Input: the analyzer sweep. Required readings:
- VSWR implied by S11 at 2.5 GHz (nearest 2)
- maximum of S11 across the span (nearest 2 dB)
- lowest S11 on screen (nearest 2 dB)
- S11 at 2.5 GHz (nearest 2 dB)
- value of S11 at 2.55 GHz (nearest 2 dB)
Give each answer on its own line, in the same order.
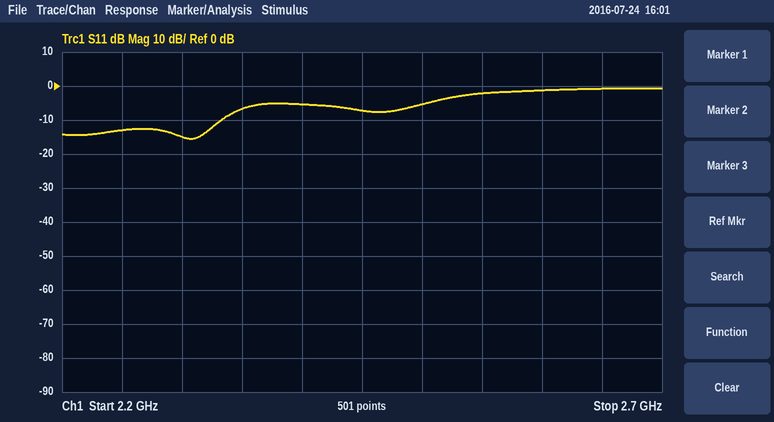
4
0 dB
-16 dB
-6 dB
-2 dB
